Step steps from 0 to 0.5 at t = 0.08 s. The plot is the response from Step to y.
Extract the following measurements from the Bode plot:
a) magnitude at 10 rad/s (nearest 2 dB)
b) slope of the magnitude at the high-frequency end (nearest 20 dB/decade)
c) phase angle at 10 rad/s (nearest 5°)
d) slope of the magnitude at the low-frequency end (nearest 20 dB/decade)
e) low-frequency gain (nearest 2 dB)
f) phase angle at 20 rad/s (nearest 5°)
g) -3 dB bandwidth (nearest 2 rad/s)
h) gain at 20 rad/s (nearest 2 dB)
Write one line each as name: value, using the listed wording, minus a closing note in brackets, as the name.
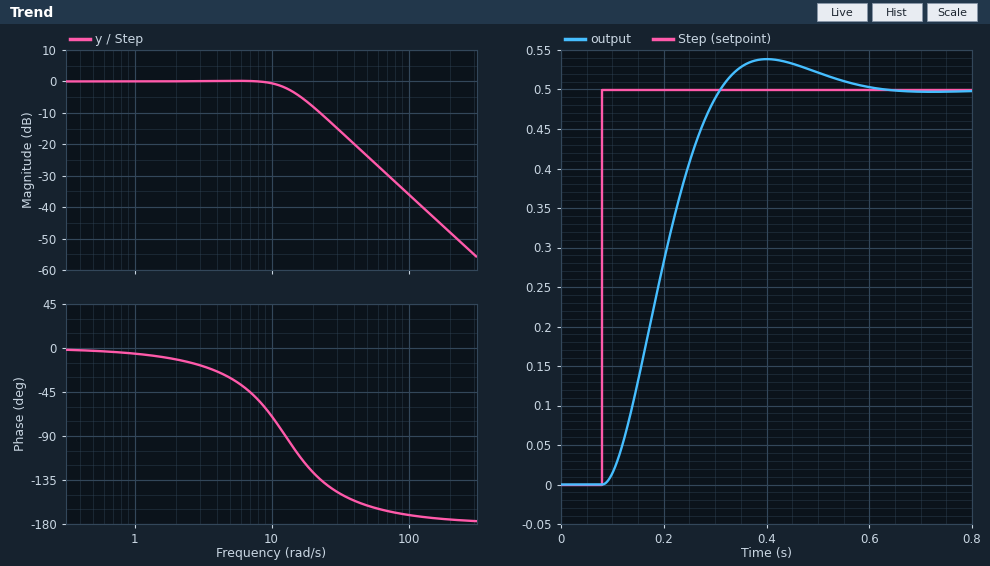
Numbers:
magnitude at 10 rad/s: 0 dB
slope of the magnitude at the high-frequency end: -40 dB/decade
phase angle at 10 rad/s: -70°
slope of the magnitude at the low-frequency end: 0 dB/decade
low-frequency gain: 0 dB
phase angle at 20 rad/s: -125°
-3 dB bandwidth: 14 rad/s
gain at 20 rad/s: -8 dB
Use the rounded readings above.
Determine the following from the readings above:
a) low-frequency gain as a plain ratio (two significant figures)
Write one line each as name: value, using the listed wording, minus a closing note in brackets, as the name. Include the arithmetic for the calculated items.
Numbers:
low-frequency gain as a plain ratio: 10^(0 / 20) = 1.0
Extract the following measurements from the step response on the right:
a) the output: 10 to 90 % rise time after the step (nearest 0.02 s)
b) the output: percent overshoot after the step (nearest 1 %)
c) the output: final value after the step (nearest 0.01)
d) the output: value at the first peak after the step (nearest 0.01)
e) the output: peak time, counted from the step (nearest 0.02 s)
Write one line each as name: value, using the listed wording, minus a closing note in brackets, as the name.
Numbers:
the output: 10 to 90 % rise time after the step: 0.16 s
the output: percent overshoot after the step: 8 %
the output: final value after the step: 0.50
the output: value at the first peak after the step: 0.54
the output: peak time, counted from the step: 0.32 s
